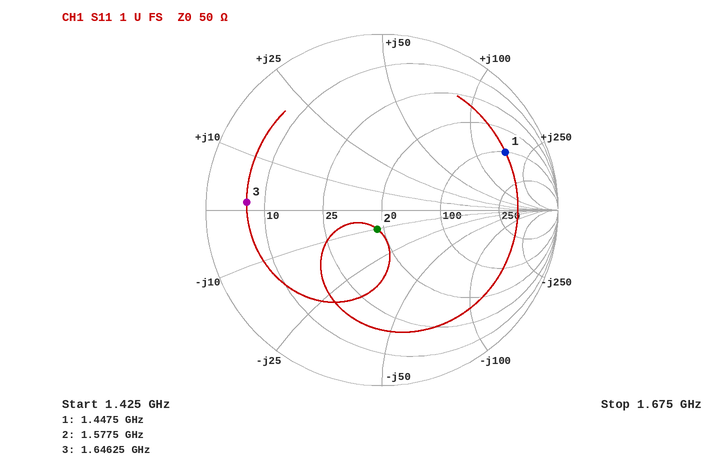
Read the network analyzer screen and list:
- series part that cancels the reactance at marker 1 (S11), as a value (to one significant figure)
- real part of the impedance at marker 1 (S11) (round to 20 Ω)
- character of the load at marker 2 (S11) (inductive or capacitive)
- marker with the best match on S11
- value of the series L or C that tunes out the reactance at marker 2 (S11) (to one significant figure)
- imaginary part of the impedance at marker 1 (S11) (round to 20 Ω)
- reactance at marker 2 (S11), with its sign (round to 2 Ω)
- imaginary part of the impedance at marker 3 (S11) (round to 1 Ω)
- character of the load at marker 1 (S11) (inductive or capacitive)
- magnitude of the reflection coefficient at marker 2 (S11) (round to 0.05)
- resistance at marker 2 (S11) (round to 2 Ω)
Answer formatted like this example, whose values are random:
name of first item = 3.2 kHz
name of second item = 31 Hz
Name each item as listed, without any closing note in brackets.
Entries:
series part that cancels the reactance at marker 1 (S11), as a value = 700 fF
real part of the impedance at marker 1 (S11) = 100 Ω
character of the load at marker 2 (S11) = capacitive
marker with the best match on S11 = marker 2
value of the series L or C that tunes out the reactance at marker 2 (S11) = 1 nH
imaginary part of the impedance at marker 1 (S11) = +160 Ω
reactance at marker 2 (S11), with its sign = -10 Ω
imaginary part of the impedance at marker 3 (S11) = +1 Ω
character of the load at marker 1 (S11) = inductive
magnitude of the reflection coefficient at marker 2 (S11) = 0.10
resistance at marker 2 (S11) = 46 Ω
